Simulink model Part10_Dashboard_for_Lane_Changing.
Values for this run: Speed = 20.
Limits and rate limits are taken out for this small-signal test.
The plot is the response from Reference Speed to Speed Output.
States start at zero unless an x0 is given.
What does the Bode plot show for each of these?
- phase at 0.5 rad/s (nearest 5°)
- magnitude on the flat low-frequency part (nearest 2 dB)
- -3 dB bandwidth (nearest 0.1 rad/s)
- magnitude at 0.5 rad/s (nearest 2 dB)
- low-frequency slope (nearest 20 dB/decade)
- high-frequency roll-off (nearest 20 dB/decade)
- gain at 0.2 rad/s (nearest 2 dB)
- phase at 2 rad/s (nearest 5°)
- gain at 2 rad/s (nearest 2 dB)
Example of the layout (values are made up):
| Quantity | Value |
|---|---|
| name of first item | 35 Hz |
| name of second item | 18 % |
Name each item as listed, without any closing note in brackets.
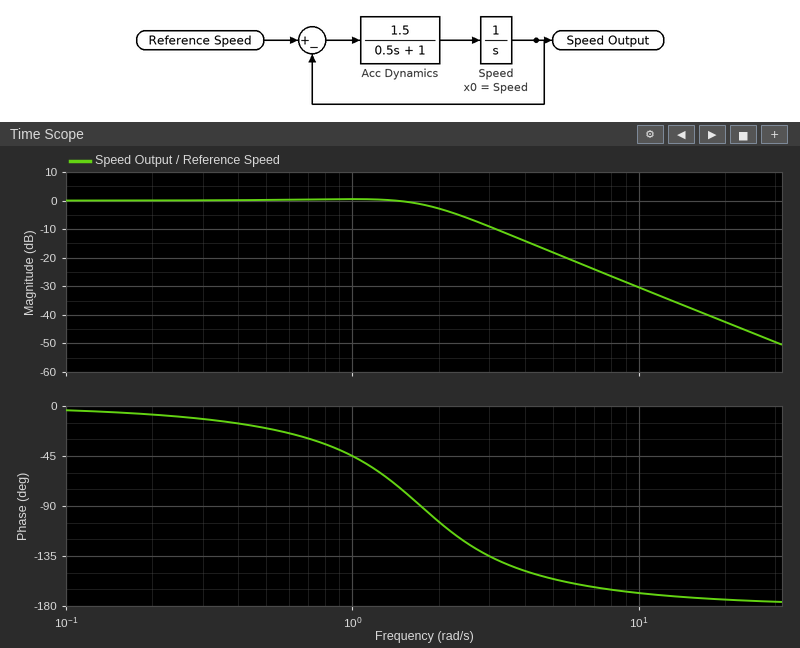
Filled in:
| Quantity | Value |
|---|---|
| phase at 0.5 rad/s | -20° |
| magnitude on the flat low-frequency part | 0 dB |
| -3 dB bandwidth | 2.0 rad/s |
| magnitude at 0.5 rad/s | 0 dB |
| low-frequency slope | 0 dB/decade |
| high-frequency roll-off | -40 dB/decade |
| gain at 0.2 rad/s | 0 dB |
| phase at 2 rad/s | -105° |
| gain at 2 rad/s | -2 dB |
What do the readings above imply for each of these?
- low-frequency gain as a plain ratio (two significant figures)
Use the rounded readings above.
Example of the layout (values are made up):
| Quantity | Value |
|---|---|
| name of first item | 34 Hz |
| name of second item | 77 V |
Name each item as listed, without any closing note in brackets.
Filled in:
| Quantity | Value |
|---|---|
| low-frequency gain as a plain ratio | 1.0 |
